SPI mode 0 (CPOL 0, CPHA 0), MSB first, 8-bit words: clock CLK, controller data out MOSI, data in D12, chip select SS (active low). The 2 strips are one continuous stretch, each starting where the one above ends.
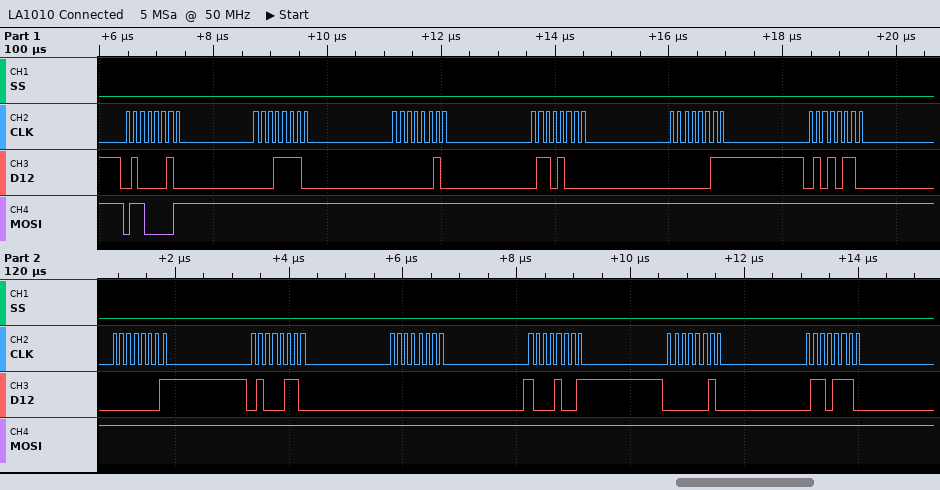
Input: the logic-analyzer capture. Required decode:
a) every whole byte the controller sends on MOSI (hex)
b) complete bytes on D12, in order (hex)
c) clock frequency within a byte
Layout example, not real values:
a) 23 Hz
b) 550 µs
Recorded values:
a) 61 FF FF FF FF FF FF FF FF FF FF FF
b) 42 1E 02 68 03 56 01 46 00 89 02 6E
c) 8 MHz
